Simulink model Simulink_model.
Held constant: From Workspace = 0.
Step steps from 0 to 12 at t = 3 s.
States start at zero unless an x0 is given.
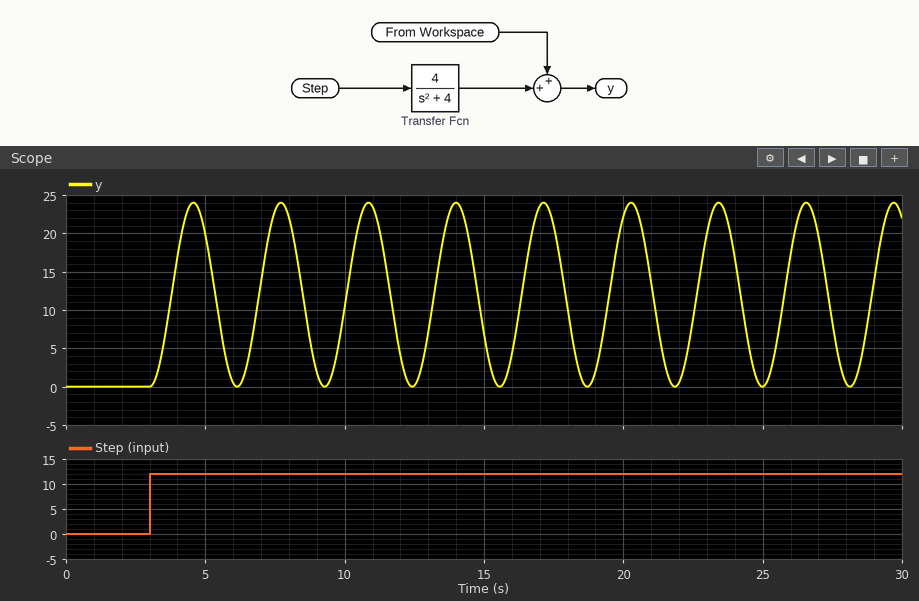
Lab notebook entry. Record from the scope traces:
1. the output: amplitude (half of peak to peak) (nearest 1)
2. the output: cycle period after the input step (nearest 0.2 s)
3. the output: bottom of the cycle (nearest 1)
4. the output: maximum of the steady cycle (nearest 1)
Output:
12
3.2 s
0
24
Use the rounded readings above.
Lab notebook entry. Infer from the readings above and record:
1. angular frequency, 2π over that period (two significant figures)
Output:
2.0 rad/s
